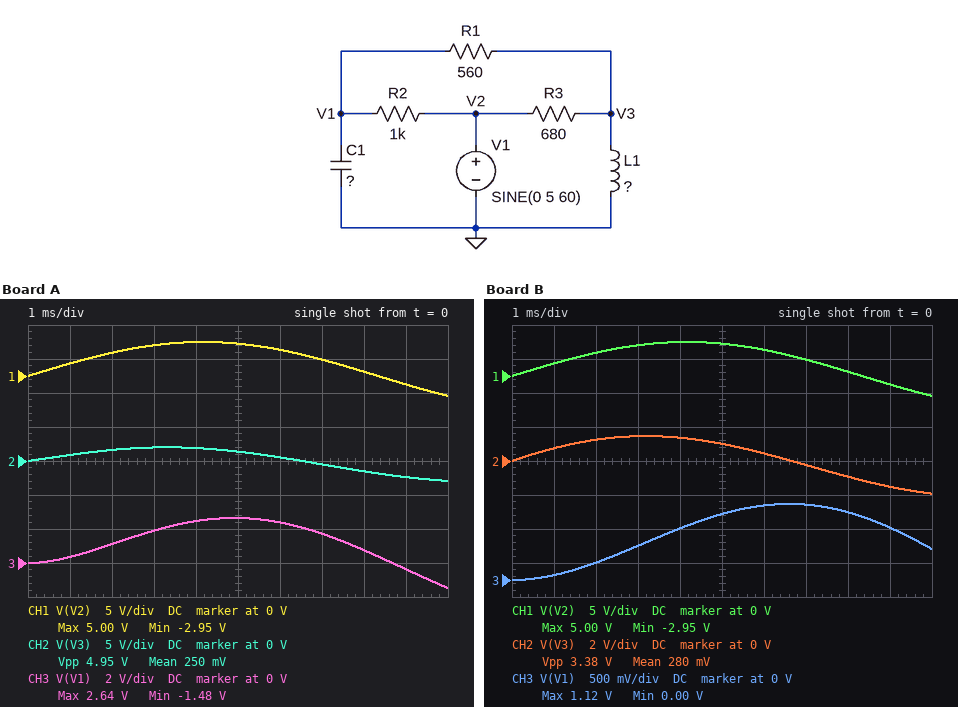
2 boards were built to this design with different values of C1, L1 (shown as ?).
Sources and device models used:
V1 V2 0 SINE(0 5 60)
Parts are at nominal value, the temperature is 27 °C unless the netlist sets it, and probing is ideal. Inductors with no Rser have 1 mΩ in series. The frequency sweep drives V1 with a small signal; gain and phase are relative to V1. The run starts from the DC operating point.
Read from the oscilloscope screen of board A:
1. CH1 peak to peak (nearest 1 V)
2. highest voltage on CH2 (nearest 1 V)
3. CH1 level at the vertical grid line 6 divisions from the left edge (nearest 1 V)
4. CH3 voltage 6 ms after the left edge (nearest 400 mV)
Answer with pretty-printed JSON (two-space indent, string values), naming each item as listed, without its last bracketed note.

{
  "CH1 peak to peak": "8 V",
  "highest voltage on CH2": "2 V",
  "CH1 level at the vertical grid line 6 divisions from the left edge": "4 V",
  "CH3 voltage 6 ms after the left edge": "2.4 V"
}
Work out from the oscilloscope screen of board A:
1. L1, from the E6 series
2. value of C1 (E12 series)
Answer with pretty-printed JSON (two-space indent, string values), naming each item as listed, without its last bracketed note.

{
  "L1, from the E6 series": "1 H",
  "value of C1": "3.9 µF"
}
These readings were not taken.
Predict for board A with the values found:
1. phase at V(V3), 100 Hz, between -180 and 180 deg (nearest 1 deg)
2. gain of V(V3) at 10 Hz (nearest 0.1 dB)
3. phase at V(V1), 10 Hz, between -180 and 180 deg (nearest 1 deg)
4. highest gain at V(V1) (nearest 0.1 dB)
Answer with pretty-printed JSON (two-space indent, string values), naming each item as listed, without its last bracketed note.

{
  "phase at V(V3), 100 Hz, between -180 and 180 deg": "12 deg",
  "gain of V(V3) at 10 Hz": "-17.6 dB",
  "phase at V(V1), 10 Hz, between -180 and 180 deg": "8 deg",
  "highest gain at V(V1)": "-3.8 dB"
}
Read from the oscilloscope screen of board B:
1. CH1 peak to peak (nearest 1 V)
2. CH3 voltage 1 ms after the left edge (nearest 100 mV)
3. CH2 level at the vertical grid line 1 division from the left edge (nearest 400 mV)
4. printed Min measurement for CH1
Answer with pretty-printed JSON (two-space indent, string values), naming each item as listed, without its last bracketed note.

{
  "CH1 peak to peak": "8 V",
  "CH3 voltage 1 ms after the left edge": "100 mV",
  "CH2 level at the vertical grid line 1 division from the left edge": "800 mV",
  "printed Min measurement for CH1": "-2.95 V"
}
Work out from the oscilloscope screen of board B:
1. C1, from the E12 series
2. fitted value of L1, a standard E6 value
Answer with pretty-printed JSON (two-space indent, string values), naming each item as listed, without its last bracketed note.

{
  "C1, from the E12 series": "22 µF",
  "fitted value of L1, a standard E6 value": "1 H"
}
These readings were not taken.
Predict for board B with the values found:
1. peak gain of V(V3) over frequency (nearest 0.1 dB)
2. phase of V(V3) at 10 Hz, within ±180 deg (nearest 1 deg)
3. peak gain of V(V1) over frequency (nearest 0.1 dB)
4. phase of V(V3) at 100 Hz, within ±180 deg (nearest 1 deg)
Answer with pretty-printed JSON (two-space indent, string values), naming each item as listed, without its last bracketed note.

{
  "peak gain of V(V3) over frequency": "-6.9 dB",
  "phase of V(V3) at 10 Hz, within ±180 deg": "74 deg",
  "peak gain of V(V1) over frequency": "-8.9 dB",
  "phase of V(V3) at 100 Hz, within ±180 deg": "18 deg"
}
